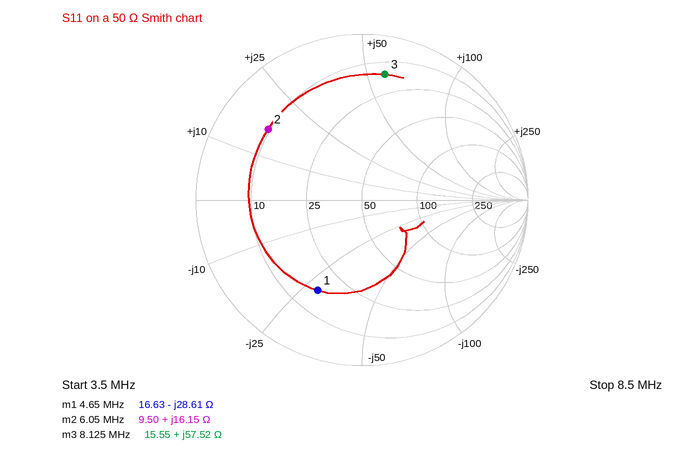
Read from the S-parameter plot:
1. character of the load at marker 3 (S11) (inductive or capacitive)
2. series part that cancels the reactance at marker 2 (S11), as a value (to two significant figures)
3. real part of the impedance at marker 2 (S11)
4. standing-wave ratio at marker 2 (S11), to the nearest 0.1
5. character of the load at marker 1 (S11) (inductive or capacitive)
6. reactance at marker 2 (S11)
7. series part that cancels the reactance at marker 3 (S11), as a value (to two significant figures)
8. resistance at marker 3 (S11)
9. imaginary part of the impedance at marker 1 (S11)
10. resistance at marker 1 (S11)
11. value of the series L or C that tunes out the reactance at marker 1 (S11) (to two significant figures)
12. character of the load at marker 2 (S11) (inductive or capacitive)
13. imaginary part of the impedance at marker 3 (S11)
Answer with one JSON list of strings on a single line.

["inductive", "1.6 nF", "9.50 Ω", "5.8", "capacitive", "+16.15 Ω", "340 pF", "15.55 Ω", "-28.61 Ω", "16.63 Ω", "980 nH", "inductive", "+57.52 Ω"]
